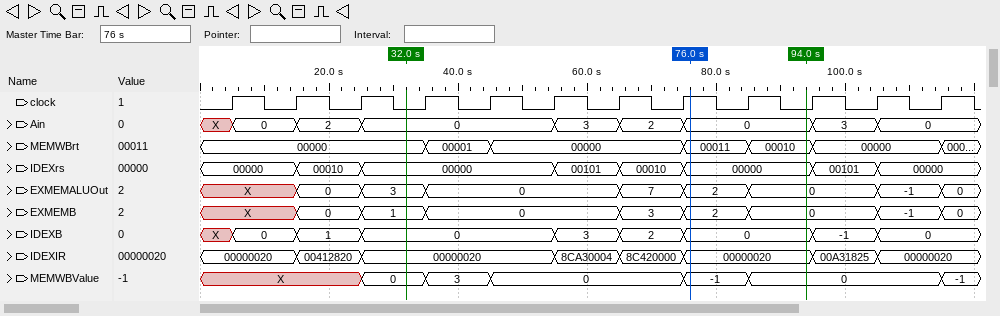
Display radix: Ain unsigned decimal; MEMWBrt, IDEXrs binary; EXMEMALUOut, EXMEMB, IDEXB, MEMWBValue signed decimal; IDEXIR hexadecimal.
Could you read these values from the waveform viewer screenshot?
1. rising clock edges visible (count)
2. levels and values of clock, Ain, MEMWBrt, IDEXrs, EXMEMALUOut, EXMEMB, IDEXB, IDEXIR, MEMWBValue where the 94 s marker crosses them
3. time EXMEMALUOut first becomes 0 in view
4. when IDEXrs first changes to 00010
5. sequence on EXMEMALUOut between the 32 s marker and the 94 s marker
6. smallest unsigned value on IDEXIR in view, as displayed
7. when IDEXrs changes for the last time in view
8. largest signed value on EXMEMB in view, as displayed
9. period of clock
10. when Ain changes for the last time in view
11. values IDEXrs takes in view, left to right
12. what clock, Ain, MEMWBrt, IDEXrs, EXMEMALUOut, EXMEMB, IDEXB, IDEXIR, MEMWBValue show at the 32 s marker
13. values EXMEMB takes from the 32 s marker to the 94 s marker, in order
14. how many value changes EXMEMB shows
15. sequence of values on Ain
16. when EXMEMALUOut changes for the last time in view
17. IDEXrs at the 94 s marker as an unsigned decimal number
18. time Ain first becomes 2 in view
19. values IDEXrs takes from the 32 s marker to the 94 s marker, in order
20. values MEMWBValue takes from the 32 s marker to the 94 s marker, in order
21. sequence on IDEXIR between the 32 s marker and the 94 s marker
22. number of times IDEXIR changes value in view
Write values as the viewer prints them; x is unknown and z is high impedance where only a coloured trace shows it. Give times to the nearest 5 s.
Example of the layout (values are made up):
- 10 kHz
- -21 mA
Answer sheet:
- 12
- clock=0, Ain=0, MEMWBrt=00010, IDEXrs=00000, EXMEMALUOut=0, EXMEMB=0, IDEXB=0, IDEXIR=00000020, MEMWBValue=0
- 15 s
- 15 s
- 3, 0, 7, 2, 0
- 00000020
- 105 s
- 3
- 10 s
- 105 s
- 00000, 00010, 00000, 00101, 00010, 00000, 00101, 00000
- clock=0, Ain=0, MEMWBrt=00000, IDEXrs=00000, EXMEMALUOut=3, EXMEMB=1, IDEXB=0, IDEXIR=00000020, MEMWBValue=0
- 1, 0, 3, 2, 0
- 8
- X, 0, 2, 0, 3, 2, 0, 3, 0
- 115 s
- 0
- 15 s
- 00000, 00101, 00010, 00000
- 0, 3, 0, -1, 0
- 00000020, 8CA30004, 8C420000, 00000020
- 7
